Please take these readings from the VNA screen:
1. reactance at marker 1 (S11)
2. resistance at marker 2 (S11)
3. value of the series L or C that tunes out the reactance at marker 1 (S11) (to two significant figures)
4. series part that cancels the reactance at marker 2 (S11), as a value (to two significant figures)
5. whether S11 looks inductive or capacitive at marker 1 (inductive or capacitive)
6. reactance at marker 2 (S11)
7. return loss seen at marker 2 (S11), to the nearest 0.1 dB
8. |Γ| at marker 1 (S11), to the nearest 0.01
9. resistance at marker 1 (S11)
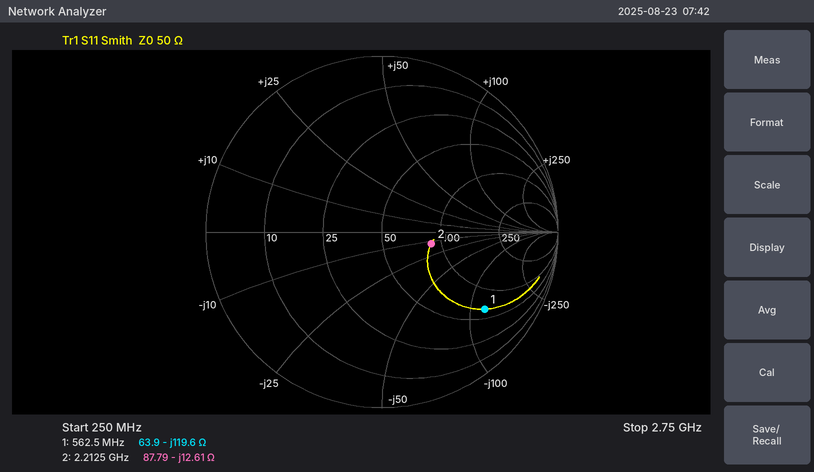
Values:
-119.6 Ω
87.79 Ω
34 nH
910 pH
capacitive
-12.61 Ω
10.8 dB
0.73
63.9 Ω
